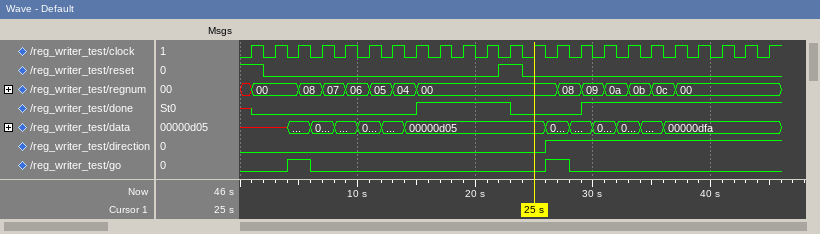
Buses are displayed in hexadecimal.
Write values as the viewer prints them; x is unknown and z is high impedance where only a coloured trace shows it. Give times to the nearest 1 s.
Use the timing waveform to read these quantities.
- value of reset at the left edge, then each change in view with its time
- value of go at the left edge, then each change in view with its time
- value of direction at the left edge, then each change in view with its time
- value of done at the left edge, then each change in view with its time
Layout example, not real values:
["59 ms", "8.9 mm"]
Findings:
["1, 0 at 2 s, 1 at 22 s, 0 at 24 s", "0, 1 at 4 s, 0 at 6 s, 1 at 26 s, 0 at 28 s", "0, 1 at 26 s", "x, 0 at 1 s, 1 at 15 s, 0 at 23 s, 1 at 29 s"]
